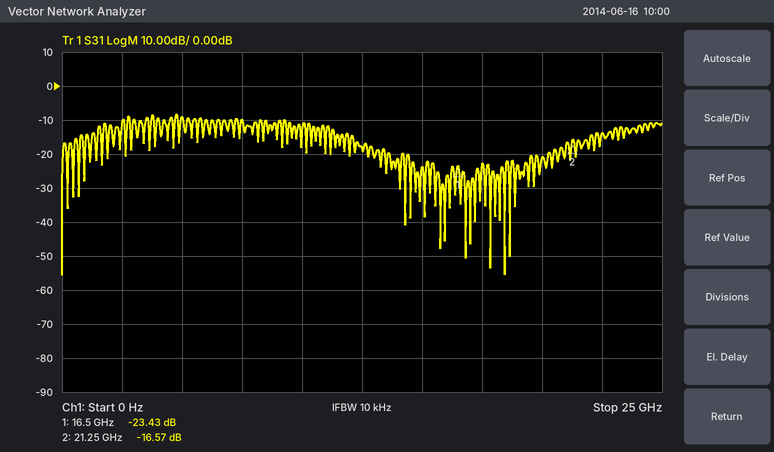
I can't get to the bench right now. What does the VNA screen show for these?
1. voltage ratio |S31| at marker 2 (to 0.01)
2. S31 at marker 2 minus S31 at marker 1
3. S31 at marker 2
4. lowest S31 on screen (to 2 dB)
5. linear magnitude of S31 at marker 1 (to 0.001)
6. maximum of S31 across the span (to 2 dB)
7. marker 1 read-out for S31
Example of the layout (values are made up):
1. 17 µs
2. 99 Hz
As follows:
1. 0.15
2. 6.86 dB
3. -16.57 dB
4. -56 dB
5. 0.067
6. -8 dB
7. -23.43 dB
